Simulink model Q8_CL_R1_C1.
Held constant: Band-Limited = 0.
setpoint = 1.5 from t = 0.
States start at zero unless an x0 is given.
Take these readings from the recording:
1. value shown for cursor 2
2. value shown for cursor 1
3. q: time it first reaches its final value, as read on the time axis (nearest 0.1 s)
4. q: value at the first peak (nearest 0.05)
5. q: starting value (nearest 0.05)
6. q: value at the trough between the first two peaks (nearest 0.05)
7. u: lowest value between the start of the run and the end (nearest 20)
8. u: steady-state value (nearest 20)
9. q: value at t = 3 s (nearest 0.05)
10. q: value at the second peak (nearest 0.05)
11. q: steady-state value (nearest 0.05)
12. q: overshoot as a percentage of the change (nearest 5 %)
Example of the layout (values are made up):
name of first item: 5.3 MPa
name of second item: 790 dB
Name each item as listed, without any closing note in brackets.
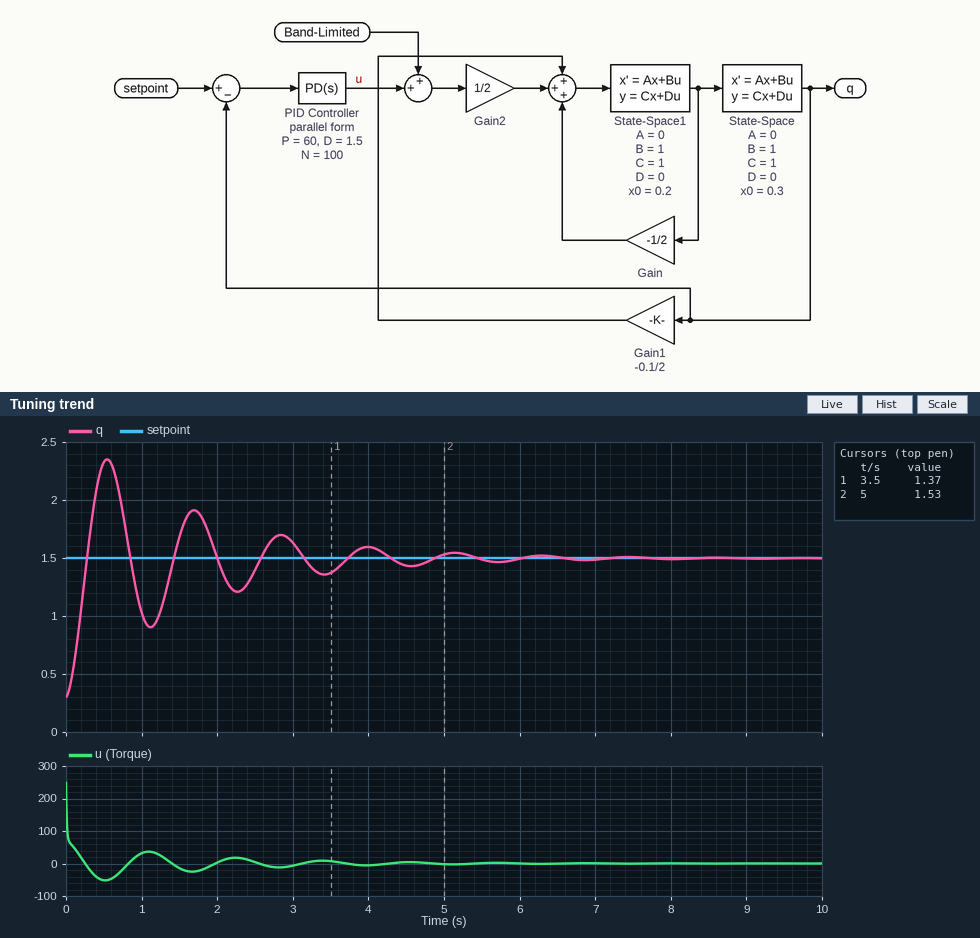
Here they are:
value shown for cursor 2: 1.53
value shown for cursor 1: 1.37
q: time it first reaches its final value, as read on the time axis: 0.3 s
q: value at the first peak: 2.35
q: starting value: 0.30
q: value at the trough between the first two peaks: 0.90
u: lowest value between the start of the run and the end: -60
u: steady-state value: 0
q: value at t = 3 s: 1.65
q: value at the second peak: 1.90
q: steady-state value: 1.50
q: overshoot as a percentage of the change: 70 %
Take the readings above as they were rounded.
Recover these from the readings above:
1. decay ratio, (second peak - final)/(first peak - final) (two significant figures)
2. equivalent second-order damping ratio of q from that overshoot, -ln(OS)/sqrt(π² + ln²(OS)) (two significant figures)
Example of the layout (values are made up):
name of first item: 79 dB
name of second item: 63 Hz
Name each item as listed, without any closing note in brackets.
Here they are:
decay ratio, (second peak - final)/(first peak - final): 0.47
equivalent second-order damping ratio of q from that overshoot, -ln(OS)/sqrt(π² + ln²(OS)): 0.11
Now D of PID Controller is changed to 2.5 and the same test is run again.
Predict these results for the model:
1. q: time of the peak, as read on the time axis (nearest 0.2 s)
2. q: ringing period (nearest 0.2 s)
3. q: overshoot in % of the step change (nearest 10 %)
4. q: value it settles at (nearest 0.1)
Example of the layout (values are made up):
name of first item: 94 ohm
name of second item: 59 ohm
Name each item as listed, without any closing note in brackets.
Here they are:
q: time of the peak, as read on the time axis: 0.6 s
q: ringing period: 1.2 s
q: overshoot in % of the step change: 60 %
q: value it settles at: 1.5
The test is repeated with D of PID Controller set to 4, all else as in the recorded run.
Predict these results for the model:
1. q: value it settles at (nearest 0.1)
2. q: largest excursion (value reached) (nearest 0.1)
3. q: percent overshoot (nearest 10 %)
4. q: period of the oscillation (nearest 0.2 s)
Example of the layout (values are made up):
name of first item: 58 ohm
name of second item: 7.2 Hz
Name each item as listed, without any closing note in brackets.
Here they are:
q: value it settles at: 1.5
q: largest excursion (value reached): 2.1
q: percent overshoot: 50 %
q: period of the oscillation: 1.2 s
